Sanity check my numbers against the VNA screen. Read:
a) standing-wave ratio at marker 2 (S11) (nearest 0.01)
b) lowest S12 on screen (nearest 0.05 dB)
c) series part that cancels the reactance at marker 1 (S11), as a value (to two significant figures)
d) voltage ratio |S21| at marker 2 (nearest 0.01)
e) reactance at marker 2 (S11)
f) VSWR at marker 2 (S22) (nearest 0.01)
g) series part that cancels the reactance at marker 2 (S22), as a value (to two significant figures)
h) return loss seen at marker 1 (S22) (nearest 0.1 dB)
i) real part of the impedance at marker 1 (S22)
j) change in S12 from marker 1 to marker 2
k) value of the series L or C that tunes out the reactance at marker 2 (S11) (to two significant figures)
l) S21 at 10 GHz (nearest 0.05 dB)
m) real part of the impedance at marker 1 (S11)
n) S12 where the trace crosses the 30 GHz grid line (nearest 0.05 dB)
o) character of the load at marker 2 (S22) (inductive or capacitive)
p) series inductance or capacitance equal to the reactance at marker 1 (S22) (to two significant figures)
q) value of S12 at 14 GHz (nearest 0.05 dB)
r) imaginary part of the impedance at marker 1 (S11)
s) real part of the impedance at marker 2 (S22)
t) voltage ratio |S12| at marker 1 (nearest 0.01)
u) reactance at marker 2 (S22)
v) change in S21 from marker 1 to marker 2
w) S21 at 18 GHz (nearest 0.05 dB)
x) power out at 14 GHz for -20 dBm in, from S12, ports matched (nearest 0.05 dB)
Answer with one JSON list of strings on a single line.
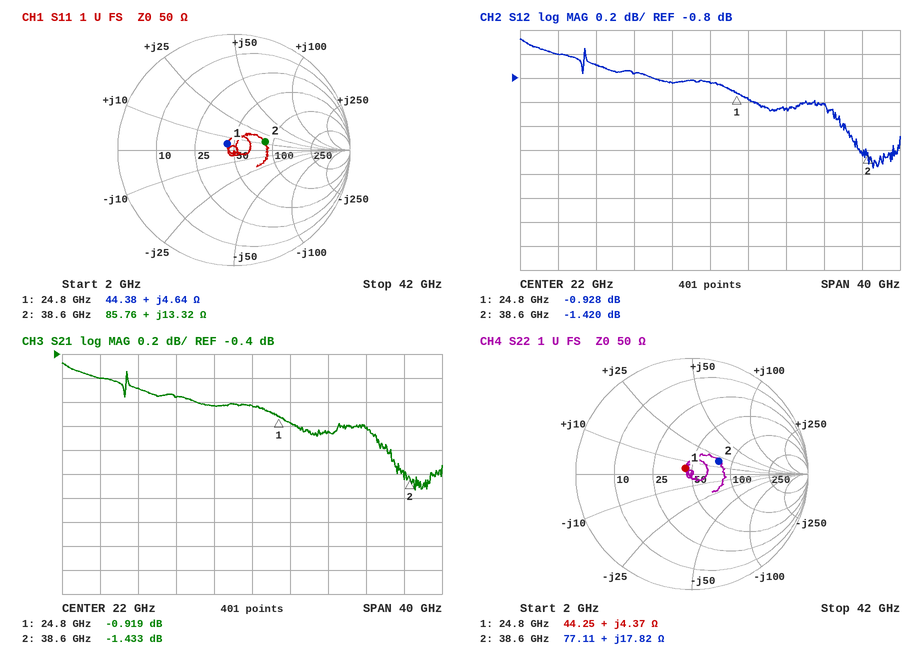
["1.78", "-1.55 dB", "1.4 pF", "0.85", "+13.32 Ω", "1.68", "230 fF", "22.3 dB", "44.25 Ω", "-0.492 dB", "310 fF", "-0.70 dB", "44.38 Ω", "-1.05 dB", "inductive", "28 pH", "-0.75 dB", "+4.64 Ω", "77.11 Ω", "0.90", "+17.82 Ω", "-0.514 dB", "-0.85 dB", "-20.75 dBm"]
